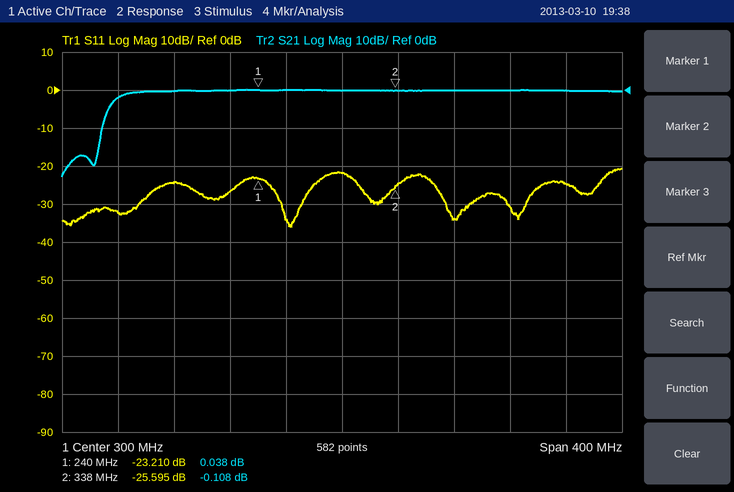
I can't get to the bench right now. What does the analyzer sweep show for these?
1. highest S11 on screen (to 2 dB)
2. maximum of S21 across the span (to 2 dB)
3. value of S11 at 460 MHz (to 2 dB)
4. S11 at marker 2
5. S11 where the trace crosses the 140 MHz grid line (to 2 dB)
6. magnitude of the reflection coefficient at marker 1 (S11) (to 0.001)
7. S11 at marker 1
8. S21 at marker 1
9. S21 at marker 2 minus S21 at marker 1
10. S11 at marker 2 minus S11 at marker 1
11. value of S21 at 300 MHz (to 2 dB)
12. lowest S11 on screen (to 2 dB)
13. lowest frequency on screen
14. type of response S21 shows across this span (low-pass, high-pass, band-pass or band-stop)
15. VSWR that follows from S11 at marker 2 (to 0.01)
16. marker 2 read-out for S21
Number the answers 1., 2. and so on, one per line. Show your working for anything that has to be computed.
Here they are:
1. -20 dB
2. 0 dB
3. -24 dB
4. -25.595 dB
5. -32 dB
6. 10^(-23.21/20) ≈ 0.069
7. -23.210 dB
8. 0.038 dB
9. -0.108 − (0.038) = -0.146 dB
10. -25.595 − (-23.21) = -2.385 dB
11. 0 dB
12. -36 dB
13. 100 MHz
14. high-pass
15. (1 + 0.0525)/(1 − 0.0525) ≈ 1.11
16. -0.108 dB
